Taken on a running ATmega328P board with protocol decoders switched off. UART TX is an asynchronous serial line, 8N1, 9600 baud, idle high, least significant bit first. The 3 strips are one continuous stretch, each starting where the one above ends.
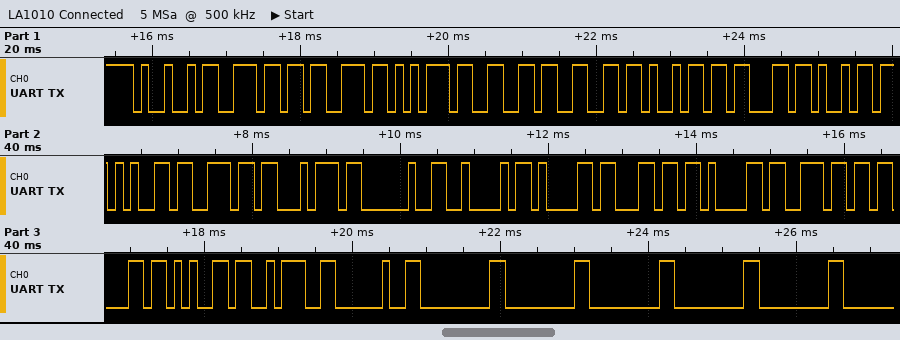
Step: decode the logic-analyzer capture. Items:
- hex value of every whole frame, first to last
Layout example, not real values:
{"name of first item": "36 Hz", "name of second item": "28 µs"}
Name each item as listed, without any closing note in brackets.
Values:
{"hex value of every whole frame, first to last": "49 6E 73 75 66 66 69 63 69 65 6E 74 20 42 61 6C 61 6E 63 65 3A 20 00 00 00 00 00"}
